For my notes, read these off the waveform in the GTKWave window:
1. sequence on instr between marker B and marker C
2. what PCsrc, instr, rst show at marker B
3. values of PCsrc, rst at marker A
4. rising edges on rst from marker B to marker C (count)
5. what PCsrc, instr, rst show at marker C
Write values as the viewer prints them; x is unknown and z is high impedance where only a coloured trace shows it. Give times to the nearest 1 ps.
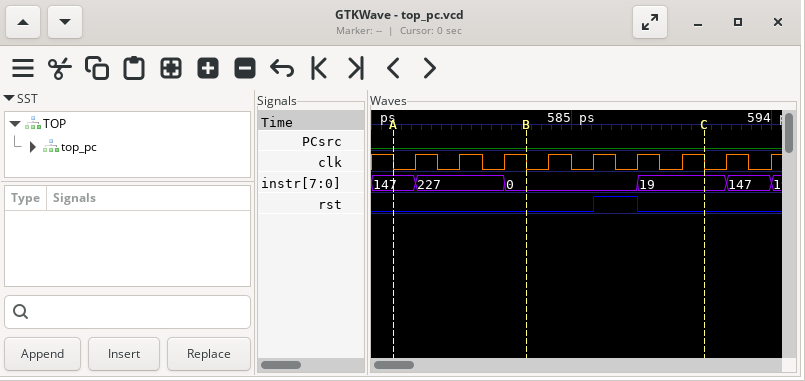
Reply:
0, 19
PCsrc=0, instr=0, rst=0
PCsrc=0, rst=0
1
PCsrc=0, instr=19, rst=0
